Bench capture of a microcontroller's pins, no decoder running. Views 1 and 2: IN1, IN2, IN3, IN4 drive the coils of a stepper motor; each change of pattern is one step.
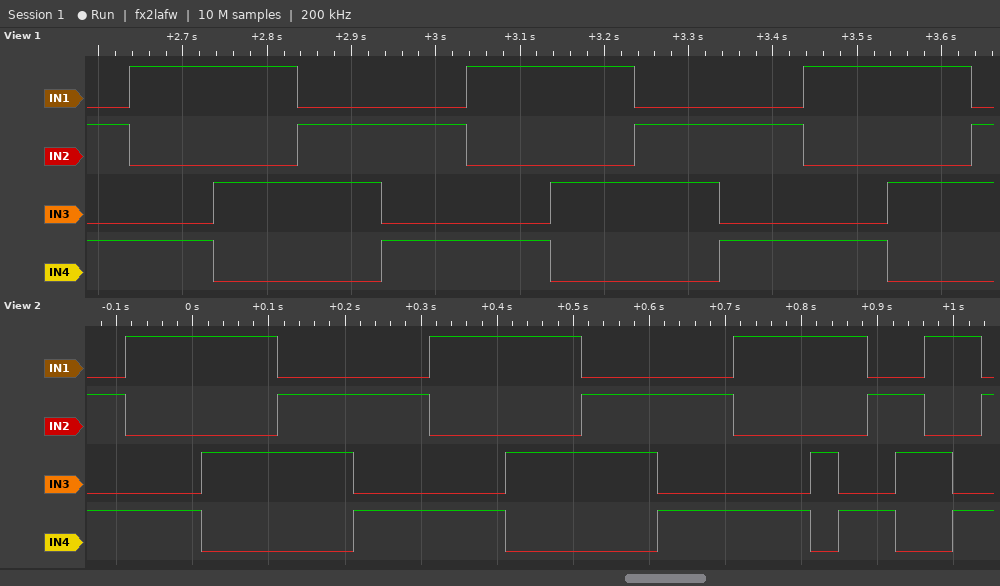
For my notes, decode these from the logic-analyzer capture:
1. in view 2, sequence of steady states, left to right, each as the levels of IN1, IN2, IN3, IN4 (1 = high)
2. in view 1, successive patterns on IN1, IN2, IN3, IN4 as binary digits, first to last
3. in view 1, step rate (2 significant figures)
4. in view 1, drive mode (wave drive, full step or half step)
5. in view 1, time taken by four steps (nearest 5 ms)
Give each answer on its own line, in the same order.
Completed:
0101 1001 1010 0110 0101 1001 1010 0110 0101 1001 1010 1001 0101 0110 1010 1001 0101
0101 1001 1010 0110 0101 1001 1010 0110 0101 1001 1010 0110
10.0 steps/s
full step
400 ms
